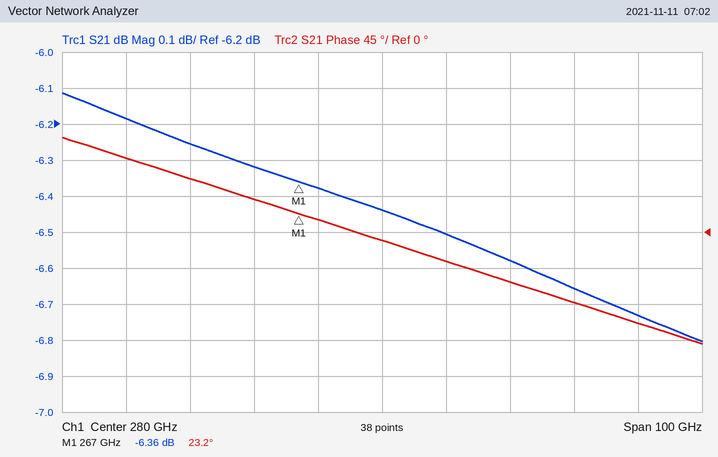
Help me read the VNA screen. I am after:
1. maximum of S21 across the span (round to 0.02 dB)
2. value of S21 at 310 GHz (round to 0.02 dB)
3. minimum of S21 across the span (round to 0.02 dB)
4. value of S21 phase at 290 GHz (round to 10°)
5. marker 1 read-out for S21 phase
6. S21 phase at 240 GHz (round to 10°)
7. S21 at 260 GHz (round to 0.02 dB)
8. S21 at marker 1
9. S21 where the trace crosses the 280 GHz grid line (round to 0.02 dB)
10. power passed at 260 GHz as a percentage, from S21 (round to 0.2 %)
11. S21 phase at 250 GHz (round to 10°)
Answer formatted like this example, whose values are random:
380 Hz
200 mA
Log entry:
-6.12 dB
-6.66 dB
-6.80 dB
-40°
23.2°
90°
-6.32 dB
-6.36 dB
-6.44 dB
23.4 %
70°
